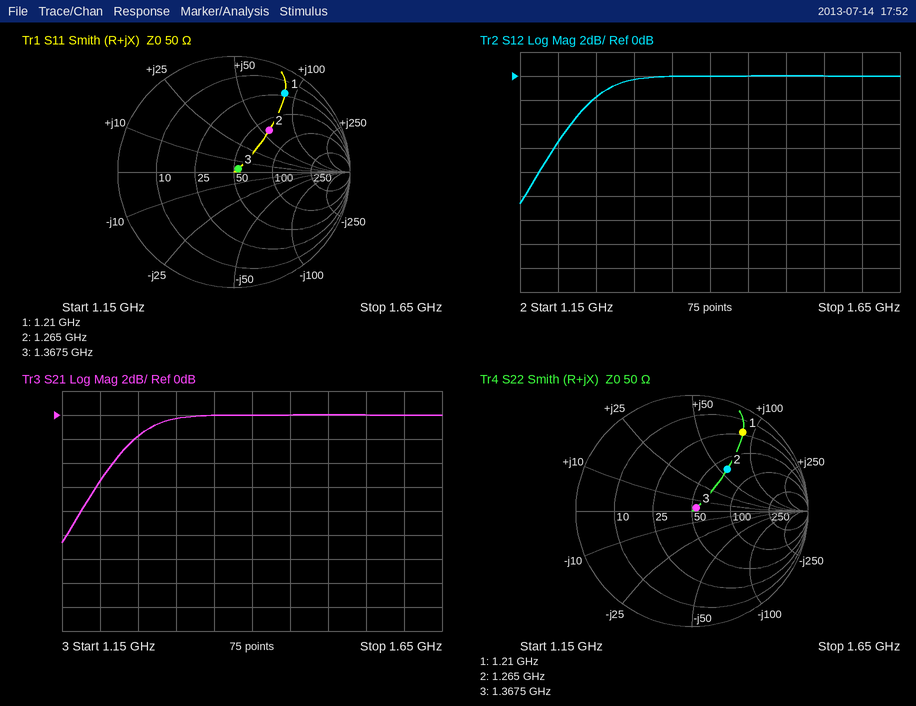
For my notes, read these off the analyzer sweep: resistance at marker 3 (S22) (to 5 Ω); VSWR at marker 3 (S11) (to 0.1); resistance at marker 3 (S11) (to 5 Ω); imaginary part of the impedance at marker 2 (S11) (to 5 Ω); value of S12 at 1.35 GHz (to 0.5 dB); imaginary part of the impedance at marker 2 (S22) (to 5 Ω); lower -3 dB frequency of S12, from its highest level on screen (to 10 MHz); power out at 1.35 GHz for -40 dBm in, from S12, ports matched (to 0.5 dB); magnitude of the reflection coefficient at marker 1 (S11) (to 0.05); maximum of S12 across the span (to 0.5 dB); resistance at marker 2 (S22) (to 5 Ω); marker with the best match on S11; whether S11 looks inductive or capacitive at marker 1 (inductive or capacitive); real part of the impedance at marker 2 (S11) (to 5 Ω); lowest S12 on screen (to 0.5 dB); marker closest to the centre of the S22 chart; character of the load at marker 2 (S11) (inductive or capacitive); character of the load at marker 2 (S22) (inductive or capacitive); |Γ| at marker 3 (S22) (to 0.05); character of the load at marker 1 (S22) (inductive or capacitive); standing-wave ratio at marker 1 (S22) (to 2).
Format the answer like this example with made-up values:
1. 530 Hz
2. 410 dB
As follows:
1. 55 Ω
2. 1.1
3. 55 Ω
4. +60 Ω
5. 0.0 dB
6. +60 Ω
7. 1.23 GHz
8. -40.0 dBm
9. 0.80
10. 0.0 dB
11. 65 Ω
12. marker 3
13. inductive
14. 65 Ω
15. -10.5 dB
16. marker 3
17. inductive
18. inductive
19. 0.05
20. inductive
21. 10
